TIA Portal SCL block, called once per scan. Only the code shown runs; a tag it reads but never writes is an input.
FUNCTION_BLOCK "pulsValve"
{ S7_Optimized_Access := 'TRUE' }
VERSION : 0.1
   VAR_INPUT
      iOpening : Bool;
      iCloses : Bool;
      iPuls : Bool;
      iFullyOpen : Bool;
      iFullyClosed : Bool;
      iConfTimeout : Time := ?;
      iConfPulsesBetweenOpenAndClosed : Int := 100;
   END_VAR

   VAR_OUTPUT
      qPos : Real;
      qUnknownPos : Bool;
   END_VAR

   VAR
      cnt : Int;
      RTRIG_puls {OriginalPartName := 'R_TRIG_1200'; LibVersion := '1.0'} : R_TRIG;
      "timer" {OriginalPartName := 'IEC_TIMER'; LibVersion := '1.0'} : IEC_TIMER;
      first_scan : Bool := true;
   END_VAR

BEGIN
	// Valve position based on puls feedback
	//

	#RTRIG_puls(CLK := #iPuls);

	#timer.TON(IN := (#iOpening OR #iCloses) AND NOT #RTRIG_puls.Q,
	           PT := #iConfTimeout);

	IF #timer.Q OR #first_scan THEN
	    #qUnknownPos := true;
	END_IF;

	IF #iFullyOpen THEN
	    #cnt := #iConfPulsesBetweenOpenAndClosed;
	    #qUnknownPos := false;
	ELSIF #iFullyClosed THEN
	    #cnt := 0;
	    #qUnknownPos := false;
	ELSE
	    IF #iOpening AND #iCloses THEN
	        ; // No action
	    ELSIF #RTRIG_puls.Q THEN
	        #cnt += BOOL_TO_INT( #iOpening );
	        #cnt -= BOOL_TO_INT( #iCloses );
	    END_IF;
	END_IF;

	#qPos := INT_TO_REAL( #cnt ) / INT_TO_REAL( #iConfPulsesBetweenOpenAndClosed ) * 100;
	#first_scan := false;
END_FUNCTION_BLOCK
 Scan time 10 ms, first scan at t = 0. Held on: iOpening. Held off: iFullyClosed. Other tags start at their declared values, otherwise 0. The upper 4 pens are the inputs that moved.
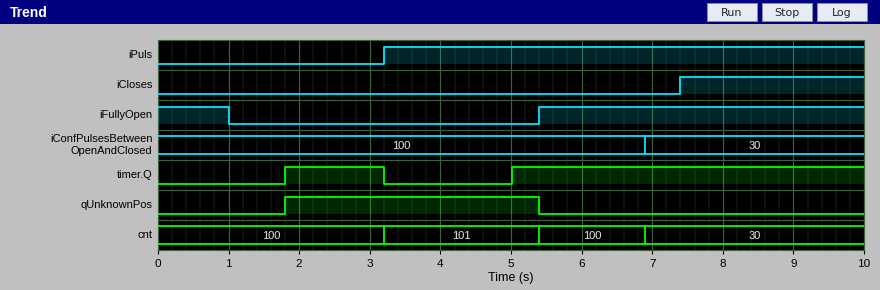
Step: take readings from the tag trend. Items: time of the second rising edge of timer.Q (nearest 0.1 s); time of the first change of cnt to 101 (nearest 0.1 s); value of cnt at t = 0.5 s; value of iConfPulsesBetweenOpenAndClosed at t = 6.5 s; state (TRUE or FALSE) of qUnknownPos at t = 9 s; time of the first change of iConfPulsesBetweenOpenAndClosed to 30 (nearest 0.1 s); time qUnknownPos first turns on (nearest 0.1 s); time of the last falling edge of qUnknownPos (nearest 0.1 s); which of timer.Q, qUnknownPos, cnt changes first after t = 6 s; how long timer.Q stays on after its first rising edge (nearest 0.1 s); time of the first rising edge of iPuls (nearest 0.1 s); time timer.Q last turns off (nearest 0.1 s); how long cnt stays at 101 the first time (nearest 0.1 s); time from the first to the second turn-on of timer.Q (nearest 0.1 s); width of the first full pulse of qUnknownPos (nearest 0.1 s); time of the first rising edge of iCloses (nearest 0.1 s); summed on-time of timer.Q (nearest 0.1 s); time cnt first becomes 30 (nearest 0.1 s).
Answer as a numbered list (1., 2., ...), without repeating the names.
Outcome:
1. 5.0 s
2. 3.2 s
3. 100
4. 100
5. FALSE
6. 6.9 s
7. 1.8 s
8. 5.4 s
9. cnt
10. 1.4 s
11. 3.2 s
12. 3.2 s
13. 2.2 s
14. 3.2 s
15. 3.6 s
16. 7.4 s
17. 6.4 s
18. 6.9 s
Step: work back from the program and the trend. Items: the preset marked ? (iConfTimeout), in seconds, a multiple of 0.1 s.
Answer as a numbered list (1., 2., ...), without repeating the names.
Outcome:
1. 1.8 s
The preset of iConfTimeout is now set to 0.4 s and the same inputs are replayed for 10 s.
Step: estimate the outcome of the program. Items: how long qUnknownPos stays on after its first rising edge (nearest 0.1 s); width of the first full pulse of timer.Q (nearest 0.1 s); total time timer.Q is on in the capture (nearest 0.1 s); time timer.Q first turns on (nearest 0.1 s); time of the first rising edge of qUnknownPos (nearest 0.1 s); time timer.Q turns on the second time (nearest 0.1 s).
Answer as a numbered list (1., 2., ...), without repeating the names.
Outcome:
1. 4.4 s
2. 2.8 s
3. 9.2 s
4. 0.4 s
5. 1.0 s
6. 3.6 s
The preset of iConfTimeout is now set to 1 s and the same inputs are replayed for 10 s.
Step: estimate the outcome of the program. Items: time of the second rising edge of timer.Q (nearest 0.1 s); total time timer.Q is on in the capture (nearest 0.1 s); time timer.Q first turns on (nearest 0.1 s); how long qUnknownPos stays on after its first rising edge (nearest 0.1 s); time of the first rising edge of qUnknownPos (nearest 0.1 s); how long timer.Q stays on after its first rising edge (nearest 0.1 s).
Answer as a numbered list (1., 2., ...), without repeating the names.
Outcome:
1. 4.2 s
2. 8.0 s
3. 1.0 s
4. 4.4 s
5. 1.0 s
6. 2.2 s
